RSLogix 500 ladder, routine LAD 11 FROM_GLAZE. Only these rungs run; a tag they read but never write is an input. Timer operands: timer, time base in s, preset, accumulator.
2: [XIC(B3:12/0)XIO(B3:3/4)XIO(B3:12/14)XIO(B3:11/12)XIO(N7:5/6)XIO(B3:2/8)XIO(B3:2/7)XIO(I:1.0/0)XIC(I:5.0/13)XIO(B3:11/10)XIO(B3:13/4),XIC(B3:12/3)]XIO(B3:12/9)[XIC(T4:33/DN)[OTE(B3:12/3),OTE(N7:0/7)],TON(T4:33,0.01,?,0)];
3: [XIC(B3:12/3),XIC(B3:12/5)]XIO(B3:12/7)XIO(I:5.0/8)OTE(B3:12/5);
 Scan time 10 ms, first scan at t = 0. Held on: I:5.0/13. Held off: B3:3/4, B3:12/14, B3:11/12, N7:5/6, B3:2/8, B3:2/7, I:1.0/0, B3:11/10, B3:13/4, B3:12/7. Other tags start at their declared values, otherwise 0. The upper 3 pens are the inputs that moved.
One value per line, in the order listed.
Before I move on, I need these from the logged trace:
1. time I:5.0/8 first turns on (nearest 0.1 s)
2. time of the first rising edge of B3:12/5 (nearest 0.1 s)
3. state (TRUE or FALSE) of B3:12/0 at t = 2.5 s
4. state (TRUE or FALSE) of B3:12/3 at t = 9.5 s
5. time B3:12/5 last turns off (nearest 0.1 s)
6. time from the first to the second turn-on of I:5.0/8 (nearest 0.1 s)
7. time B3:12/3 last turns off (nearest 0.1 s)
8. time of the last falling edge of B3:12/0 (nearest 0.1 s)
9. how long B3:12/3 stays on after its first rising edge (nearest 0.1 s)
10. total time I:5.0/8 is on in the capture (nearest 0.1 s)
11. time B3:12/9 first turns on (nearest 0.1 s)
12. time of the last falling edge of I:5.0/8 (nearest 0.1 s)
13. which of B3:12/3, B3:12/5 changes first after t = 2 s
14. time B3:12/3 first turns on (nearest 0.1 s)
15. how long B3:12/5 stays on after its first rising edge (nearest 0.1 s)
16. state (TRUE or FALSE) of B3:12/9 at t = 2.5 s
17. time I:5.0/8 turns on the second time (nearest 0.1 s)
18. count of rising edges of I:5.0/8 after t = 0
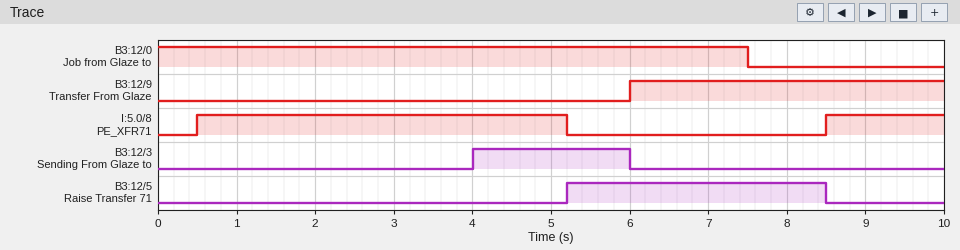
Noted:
0.5 s
5.2 s
TRUE
FALSE
8.5 s
8.0 s
6.0 s
7.5 s
2.0 s
6.2 s
6.0 s
5.2 s
B3:12/3
4.0 s
3.3 s
FALSE
8.5 s
2
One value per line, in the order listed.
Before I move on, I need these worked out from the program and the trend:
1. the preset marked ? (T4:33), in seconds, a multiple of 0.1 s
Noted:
4.0 s
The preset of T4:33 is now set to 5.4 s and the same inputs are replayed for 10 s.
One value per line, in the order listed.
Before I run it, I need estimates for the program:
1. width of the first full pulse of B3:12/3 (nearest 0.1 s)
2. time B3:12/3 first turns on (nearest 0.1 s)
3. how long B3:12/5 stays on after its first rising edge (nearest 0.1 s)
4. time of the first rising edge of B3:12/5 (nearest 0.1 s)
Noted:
0.6 s
5.4 s
3.1 s
5.4 s
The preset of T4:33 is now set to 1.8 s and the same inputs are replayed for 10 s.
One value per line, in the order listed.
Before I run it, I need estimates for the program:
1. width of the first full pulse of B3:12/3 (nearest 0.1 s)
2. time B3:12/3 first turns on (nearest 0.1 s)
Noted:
4.2 s
1.8 s
